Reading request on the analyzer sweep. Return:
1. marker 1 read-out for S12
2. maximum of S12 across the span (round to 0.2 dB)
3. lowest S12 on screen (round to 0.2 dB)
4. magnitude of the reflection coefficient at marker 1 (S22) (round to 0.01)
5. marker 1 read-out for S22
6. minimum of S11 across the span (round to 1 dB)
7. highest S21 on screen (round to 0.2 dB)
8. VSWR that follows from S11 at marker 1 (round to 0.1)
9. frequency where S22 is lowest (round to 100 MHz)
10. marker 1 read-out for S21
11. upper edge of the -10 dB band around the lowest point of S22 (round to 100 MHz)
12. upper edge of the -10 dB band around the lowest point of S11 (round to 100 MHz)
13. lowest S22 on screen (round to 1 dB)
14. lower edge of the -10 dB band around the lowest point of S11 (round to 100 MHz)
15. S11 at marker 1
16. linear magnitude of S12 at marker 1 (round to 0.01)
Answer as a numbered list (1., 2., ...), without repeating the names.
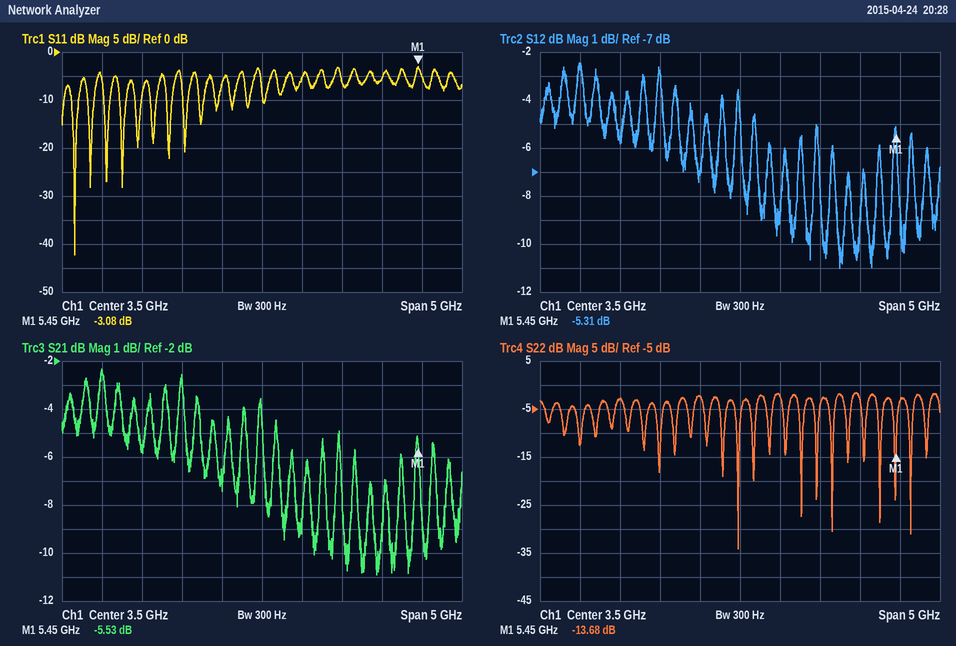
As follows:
1. -5.31 dB
2. -2.4 dB
3. -11.0 dB
4. 0.21
5. -13.68 dB
6. -42 dB
7. -2.4 dB
8. 5.7
9. 3.5 GHz
10. -5.53 dB
11. 3.5 GHz
12. 1.2 GHz
13. -34 dB
14. 1.1 GHz
15. -3.08 dB
16. 0.54
